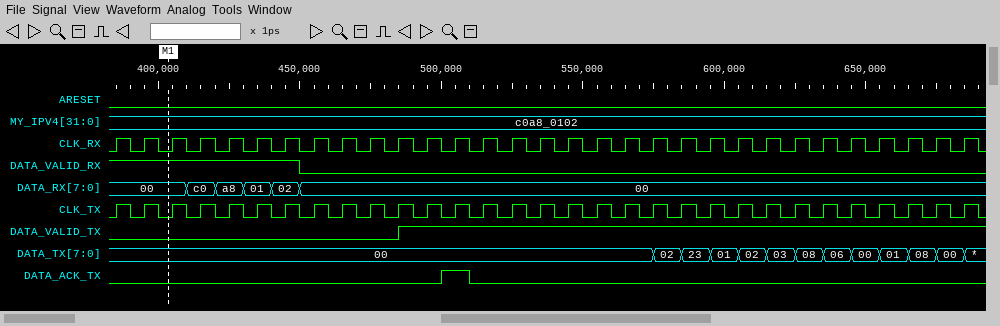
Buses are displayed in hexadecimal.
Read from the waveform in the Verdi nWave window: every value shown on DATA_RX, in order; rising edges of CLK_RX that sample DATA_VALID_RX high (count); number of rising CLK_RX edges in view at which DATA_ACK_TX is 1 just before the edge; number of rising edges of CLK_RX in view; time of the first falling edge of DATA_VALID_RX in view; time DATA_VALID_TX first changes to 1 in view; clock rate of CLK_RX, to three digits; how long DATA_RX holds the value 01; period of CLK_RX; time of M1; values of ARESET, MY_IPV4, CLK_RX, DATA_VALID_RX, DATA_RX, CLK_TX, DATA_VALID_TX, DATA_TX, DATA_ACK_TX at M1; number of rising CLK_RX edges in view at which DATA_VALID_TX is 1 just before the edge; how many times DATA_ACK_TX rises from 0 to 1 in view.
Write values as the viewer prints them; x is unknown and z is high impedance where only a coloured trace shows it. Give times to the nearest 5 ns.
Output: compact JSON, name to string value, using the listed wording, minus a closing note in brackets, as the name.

{"every value shown on DATA_RX, in order": "00, c0, a8, 01, 02, 00", "rising edges of CLK_RX that sample DATA_VALID_RX high": "7", "number of rising CLK_RX edges in view at which DATA_ACK_TX is 1 just before the edge": "1", "number of rising edges of CLK_RX in view": "31", "time of the first falling edge of DATA_VALID_RX in view": "450 ns", "time DATA_VALID_TX first changes to 1 in view": "485 ns", "clock rate of CLK_RX, to three digits": "100 MHz", "how long DATA_RX holds the value 01": "10 ns", "period of CLK_RX": "10 ns", "time of M1": "405 ns", "values of ARESET, MY_IPV4, CLK_RX, DATA_VALID_RX, DATA_RX, CLK_TX, DATA_VALID_TX, DATA_TX, DATA_ACK_TX at M1": "ARESET=0, MY_IPV4=c0a8_0102, CLK_RX=0, DATA_VALID_RX=1, DATA_RX=00, CLK_TX=0, DATA_VALID_TX=0, DATA_TX=00, DATA_ACK_TX=0", "number of rising CLK_RX edges in view at which DATA_VALID_TX is 1 just before the edge": "20", "how many times DATA_ACK_TX rises from 0 to 1 in view": "1"}
